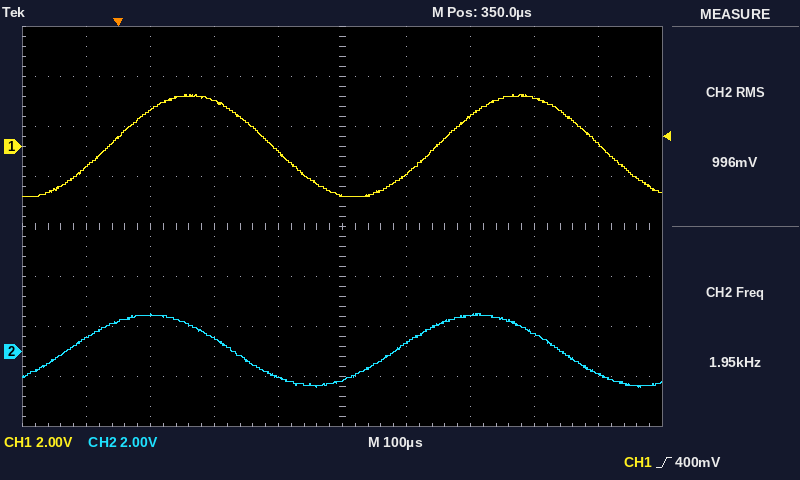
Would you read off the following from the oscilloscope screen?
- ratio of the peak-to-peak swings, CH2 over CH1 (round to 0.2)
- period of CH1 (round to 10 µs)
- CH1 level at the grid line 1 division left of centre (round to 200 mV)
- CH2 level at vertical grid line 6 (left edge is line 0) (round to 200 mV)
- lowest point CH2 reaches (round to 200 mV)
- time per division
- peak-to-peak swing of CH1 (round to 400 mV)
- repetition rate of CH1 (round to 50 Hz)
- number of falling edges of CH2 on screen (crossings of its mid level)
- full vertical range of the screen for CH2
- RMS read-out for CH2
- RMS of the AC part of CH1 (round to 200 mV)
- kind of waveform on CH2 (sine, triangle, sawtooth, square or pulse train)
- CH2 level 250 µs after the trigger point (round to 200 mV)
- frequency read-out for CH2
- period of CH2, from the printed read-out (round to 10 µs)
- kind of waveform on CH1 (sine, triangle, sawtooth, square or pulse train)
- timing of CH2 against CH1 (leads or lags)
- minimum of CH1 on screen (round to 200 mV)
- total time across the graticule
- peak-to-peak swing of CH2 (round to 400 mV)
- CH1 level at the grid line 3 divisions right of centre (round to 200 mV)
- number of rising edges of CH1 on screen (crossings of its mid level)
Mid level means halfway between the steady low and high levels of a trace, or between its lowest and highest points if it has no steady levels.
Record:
0.8
510 µs
-200 mV
400 mV
-1.4 V
100 µs
4.0 V
1.95 kHz
2
16 V
996 mV
1.4 V
sine
-1.0 V
1.95 kHz
510 µs
sine
leads
-2.0 V
1 ms
2.8 V
2.0 V
2
